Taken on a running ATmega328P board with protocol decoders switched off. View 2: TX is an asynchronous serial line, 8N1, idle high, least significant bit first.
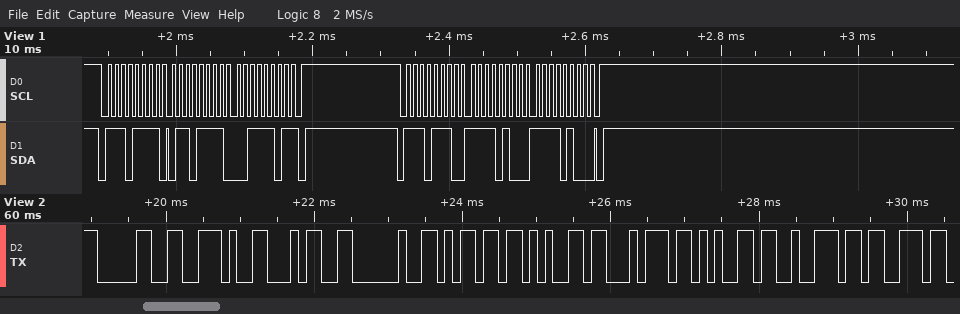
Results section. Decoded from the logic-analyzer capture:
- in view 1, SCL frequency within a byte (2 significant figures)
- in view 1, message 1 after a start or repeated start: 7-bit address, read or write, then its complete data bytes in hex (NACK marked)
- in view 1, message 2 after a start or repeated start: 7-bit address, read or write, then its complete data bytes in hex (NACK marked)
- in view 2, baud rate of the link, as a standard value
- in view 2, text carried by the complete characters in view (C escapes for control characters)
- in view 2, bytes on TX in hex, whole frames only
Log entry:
100 kHz
0x77 read: 6F 3D NACK
0x77 write: F4 F4
9600 baud
"0.4 meters"
30 2E 34 20 6D 65 74 65 72 73
